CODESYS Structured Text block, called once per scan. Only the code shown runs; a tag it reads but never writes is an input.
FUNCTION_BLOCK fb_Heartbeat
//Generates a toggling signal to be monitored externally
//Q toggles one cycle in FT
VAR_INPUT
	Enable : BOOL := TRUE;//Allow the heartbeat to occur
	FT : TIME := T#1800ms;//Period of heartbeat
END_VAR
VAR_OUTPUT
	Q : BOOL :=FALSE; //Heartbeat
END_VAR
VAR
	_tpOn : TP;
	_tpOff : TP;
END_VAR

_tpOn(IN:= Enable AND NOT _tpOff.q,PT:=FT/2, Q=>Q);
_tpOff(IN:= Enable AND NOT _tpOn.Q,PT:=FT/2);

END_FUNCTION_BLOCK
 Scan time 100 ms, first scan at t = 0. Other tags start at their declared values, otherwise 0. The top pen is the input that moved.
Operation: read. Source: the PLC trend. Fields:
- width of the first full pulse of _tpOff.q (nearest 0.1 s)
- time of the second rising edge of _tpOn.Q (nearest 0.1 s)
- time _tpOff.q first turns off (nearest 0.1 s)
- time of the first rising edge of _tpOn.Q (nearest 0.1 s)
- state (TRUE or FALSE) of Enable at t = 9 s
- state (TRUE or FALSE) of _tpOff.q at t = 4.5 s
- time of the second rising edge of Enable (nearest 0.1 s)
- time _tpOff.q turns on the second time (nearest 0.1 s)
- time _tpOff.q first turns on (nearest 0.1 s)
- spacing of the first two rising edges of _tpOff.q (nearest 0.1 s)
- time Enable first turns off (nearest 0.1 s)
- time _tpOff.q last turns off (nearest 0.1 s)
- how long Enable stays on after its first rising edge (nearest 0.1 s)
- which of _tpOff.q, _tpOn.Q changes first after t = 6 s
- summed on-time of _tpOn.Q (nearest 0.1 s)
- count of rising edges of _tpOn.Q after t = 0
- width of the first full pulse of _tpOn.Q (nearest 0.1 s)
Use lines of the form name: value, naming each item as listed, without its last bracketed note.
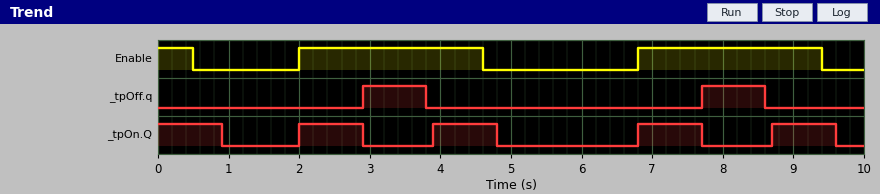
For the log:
width of the first full pulse of _tpOff.q: 0.9 s
time of the second rising edge of _tpOn.Q: 3.9 s
time _tpOff.q first turns off: 3.8 s
time of the first rising edge of _tpOn.Q: 2.0 s
state (TRUE or FALSE) of Enable at t = 9 s: TRUE
state (TRUE or FALSE) of _tpOff.q at t = 4.5 s: FALSE
time of the second rising edge of Enable: 6.8 s
time _tpOff.q turns on the second time: 7.7 s
time _tpOff.q first turns on: 2.9 s
spacing of the first two rising edges of _tpOff.q: 4.8 s
time Enable first turns off: 0.5 s
time _tpOff.q last turns off: 8.6 s
how long Enable stays on after its first rising edge: 2.6 s
which of _tpOff.q, _tpOn.Q changes first after t = 6 s: _tpOn.Q
summed on-time of _tpOn.Q: 4.5 s
count of rising edges of _tpOn.Q after t = 0: 4
width of the first full pulse of _tpOn.Q: 0.9 s
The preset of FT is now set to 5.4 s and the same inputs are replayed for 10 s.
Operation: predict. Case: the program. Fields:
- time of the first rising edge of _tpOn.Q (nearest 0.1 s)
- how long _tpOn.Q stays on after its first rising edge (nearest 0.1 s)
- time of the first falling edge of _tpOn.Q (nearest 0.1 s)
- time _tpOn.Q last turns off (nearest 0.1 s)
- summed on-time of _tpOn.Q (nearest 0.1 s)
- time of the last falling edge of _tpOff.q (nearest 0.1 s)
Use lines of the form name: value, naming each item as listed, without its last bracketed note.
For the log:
time of the first rising edge of _tpOn.Q: 6.8 s
how long _tpOn.Q stays on after its first rising edge: 2.7 s
time of the first falling edge of _tpOn.Q: 2.7 s
time _tpOn.Q last turns off: 9.5 s
summed on-time of _tpOn.Q: 5.4 s
time of the last falling edge of _tpOff.q: 5.4 s
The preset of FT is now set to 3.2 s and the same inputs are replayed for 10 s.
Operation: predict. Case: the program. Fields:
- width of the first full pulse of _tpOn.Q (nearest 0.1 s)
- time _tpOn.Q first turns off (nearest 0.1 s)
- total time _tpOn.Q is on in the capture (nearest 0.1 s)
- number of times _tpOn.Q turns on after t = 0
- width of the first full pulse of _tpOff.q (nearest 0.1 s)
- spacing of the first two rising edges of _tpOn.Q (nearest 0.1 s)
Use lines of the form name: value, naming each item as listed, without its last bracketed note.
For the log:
width of the first full pulse of _tpOn.Q: 1.6 s
time _tpOn.Q first turns off: 1.6 s
total time _tpOn.Q is on in the capture: 4.8 s
number of times _tpOn.Q turns on after t = 0: 2
width of the first full pulse of _tpOff.q: 1.6 s
spacing of the first two rising edges of _tpOn.Q: 4.8 s
